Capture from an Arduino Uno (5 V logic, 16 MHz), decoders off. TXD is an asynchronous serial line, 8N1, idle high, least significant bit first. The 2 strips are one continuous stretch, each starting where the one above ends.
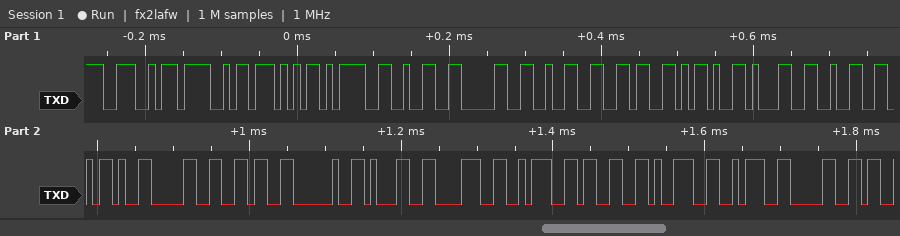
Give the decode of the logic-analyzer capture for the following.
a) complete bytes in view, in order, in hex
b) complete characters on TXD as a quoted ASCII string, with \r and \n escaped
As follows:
0x4E 0x4F 0x57 0x3D 0x32 0x30 0x32 0x36 0x2D 0x31 0x32 0x2D 0x30 0x36 0x20 0x31 0x38 0x3A 0x33 0x39 0x3A 0x30
"NOW=2026-12-06 18:39:0"
